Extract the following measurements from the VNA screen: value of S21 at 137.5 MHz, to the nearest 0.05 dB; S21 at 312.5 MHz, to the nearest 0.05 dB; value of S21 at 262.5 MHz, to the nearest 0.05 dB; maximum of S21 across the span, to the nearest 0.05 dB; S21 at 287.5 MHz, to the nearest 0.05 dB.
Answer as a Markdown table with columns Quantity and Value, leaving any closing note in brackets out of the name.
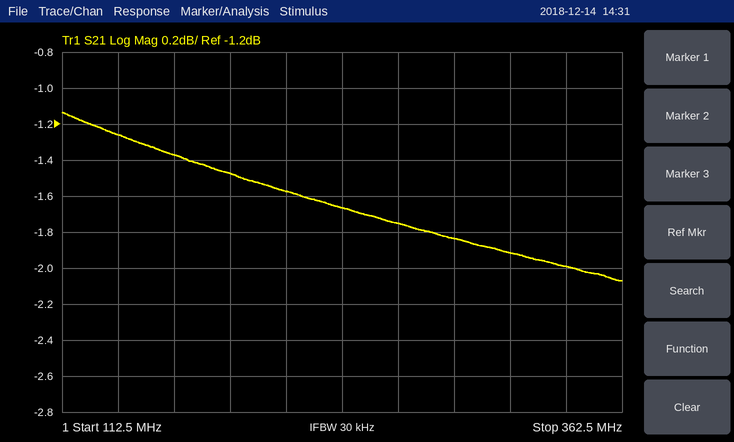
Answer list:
| Quantity | Value |
|---|---|
| value of S21 at 137.5 MHz, to the nearest 0.05 dB | -1.25 dB |
| S21 at 312.5 MHz, to the nearest 0.05 dB | -1.90 dB |
| value of S21 at 262.5 MHz, to the nearest 0.05 dB | -1.75 dB |
| maximum of S21 across the span, to the nearest 0.05 dB | -1.15 dB |
| S21 at 287.5 MHz, to the nearest 0.05 dB | -1.85 dB |
